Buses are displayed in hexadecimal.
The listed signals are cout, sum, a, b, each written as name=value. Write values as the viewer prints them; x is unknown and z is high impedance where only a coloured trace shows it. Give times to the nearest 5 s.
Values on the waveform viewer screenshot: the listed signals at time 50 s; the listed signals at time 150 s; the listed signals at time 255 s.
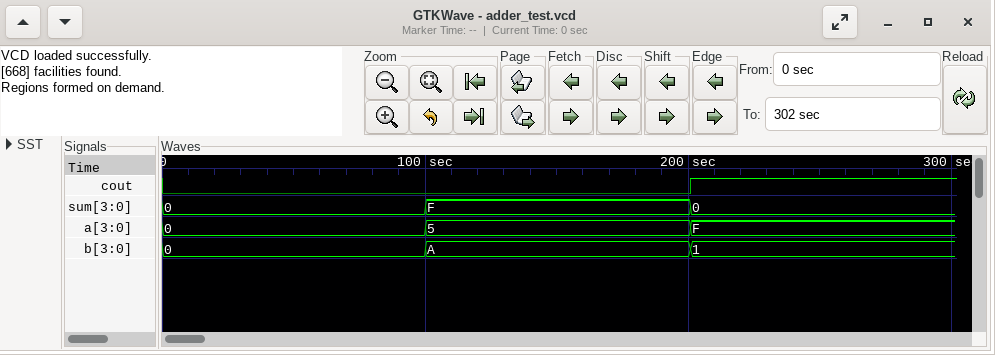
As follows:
cout=0, sum=0, a=0, b=0
cout=0, sum=F, a=5, b=A
cout=1, sum=0, a=F, b=1
